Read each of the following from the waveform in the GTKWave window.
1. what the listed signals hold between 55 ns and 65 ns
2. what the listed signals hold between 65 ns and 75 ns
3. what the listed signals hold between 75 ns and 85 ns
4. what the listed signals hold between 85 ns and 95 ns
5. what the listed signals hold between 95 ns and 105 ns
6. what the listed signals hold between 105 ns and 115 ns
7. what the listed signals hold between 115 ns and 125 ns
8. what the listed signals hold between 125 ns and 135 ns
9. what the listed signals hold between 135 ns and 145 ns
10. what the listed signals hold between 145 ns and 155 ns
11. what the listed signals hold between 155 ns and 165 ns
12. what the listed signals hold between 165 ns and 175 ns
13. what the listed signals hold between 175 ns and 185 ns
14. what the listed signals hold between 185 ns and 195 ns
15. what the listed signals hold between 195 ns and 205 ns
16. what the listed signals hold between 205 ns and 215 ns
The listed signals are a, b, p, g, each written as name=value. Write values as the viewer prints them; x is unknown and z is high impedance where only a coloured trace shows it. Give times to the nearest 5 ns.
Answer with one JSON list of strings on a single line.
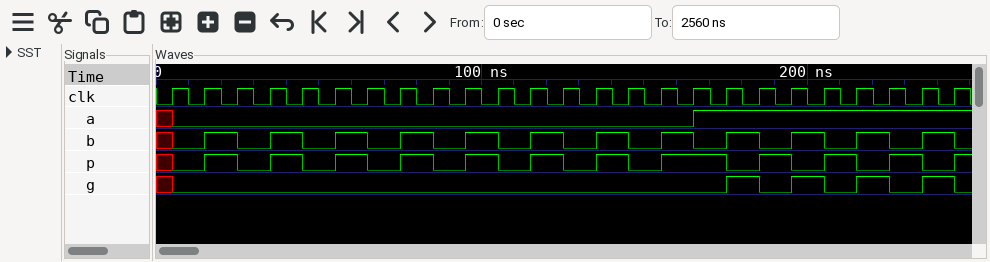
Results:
["a=0, b=1, p=1, g=0", "a=0, b=0, p=0, g=0", "a=0, b=1, p=1, g=0", "a=0, b=0, p=0, g=0", "a=0, b=1, p=1, g=0", "a=0, b=0, p=0, g=0", "a=0, b=1, p=1, g=0", "a=0, b=0, p=0, g=0", "a=0, b=1, p=1, g=0", "a=0, b=0, p=0, g=0", "a=0, b=1, p=1, g=0", "a=1, b=0, p=1, g=0", "a=1, b=1, p=0, g=1", "a=1, b=0, p=1, g=0", "a=1, b=1, p=0, g=1", "a=1, b=0, p=1, g=0"]
